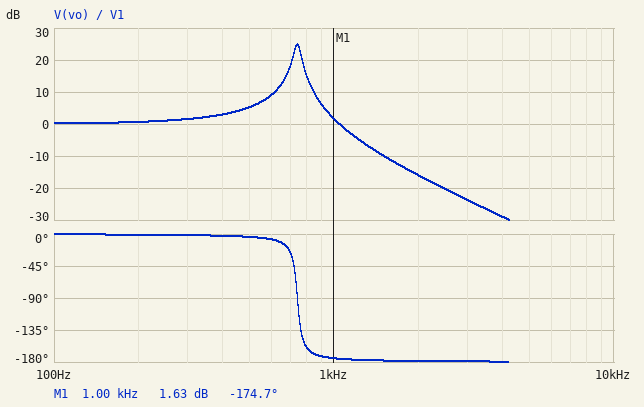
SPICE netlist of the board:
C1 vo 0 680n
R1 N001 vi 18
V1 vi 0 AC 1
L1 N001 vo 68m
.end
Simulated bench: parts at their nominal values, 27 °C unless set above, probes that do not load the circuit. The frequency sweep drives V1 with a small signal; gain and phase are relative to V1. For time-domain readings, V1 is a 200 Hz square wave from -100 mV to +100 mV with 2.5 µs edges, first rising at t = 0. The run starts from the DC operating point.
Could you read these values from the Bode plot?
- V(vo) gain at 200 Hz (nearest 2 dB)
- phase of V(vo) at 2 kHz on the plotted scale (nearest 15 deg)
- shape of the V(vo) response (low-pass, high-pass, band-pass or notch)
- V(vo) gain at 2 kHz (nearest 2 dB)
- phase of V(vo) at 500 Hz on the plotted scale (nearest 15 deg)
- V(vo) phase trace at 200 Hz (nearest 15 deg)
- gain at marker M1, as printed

0 dB
-180 deg
low-pass
-16 dB
0 deg
0 deg
1.63 dB
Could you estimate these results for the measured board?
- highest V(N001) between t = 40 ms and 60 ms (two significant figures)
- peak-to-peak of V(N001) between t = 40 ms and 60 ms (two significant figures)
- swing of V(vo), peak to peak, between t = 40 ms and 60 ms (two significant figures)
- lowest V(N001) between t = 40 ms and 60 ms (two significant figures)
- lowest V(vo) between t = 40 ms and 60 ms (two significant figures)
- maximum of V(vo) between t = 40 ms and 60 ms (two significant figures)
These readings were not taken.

110 mV
210 mV
440 mV
-110 mV
-220 mV
220 mV
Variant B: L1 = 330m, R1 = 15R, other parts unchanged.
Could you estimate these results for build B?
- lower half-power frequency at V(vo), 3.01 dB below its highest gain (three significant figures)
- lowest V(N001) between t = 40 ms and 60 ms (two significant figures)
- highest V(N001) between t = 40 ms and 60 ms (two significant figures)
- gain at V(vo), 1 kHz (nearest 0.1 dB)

332 Hz
-100 mV
100 mV
-17.9 dB
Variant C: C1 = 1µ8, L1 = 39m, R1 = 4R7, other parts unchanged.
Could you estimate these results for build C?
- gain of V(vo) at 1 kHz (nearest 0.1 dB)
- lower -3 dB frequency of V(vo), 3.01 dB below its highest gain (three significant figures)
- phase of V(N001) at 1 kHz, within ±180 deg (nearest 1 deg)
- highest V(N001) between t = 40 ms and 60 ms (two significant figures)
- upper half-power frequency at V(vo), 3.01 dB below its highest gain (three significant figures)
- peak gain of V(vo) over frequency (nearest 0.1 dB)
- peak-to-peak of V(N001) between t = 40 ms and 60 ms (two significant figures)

-5.0 dB
591 Hz
2 deg
140 mV
610 Hz
29.9 dB
280 mV
